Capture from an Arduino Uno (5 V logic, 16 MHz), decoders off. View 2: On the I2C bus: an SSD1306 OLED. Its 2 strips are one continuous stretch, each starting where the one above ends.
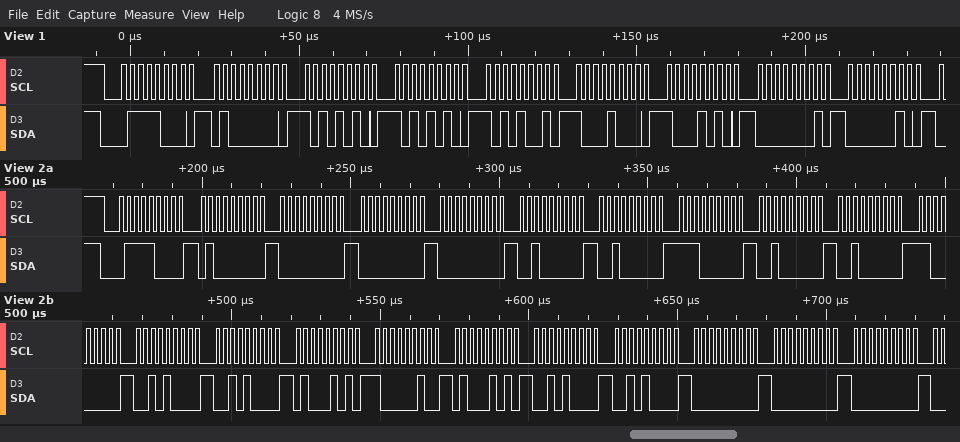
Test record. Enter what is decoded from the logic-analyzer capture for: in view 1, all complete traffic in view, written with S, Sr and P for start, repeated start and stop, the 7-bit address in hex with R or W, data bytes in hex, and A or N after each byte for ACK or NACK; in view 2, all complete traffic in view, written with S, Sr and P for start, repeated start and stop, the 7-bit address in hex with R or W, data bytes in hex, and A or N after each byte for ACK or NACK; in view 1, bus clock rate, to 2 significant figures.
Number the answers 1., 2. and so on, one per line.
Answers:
1. S 3CW A 40 A AA A AA A A9 A 88 A 8A A 01 A 02 A
2. S 3CW A 40 A 00 A 00 A 00 A 20 A 20 A E0 A 20 A 20 A C0 A 28 A 28 A 45 A 82 A 45 A 28 A 28 A 00 A 00 A 00 A
3. 400 kHz
